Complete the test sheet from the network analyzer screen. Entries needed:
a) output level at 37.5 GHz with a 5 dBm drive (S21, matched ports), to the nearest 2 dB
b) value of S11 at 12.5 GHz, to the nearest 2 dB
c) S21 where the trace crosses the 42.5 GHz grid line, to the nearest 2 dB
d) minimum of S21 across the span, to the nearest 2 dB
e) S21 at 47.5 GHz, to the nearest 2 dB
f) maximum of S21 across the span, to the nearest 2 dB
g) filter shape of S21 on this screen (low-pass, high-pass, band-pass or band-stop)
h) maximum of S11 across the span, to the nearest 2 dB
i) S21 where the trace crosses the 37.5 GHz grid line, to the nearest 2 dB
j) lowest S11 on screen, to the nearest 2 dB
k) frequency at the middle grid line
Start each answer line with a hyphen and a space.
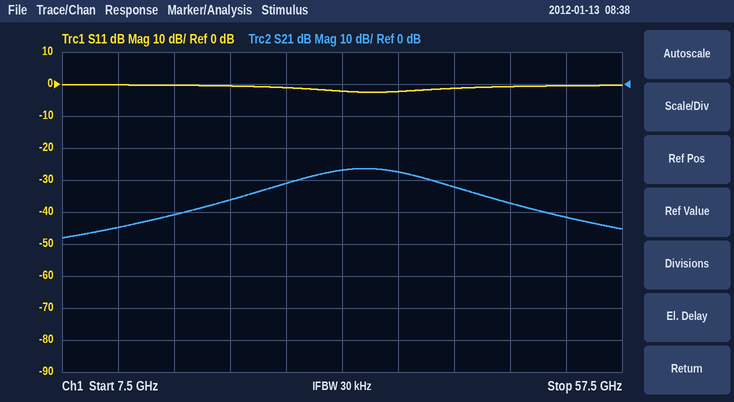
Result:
- -22 dBm
- 0 dB
- -32 dB
- -48 dB
- -38 dB
- -26 dB
- band-pass
- 0 dB
- -28 dB
- -2 dB
- 32.5 GHz
